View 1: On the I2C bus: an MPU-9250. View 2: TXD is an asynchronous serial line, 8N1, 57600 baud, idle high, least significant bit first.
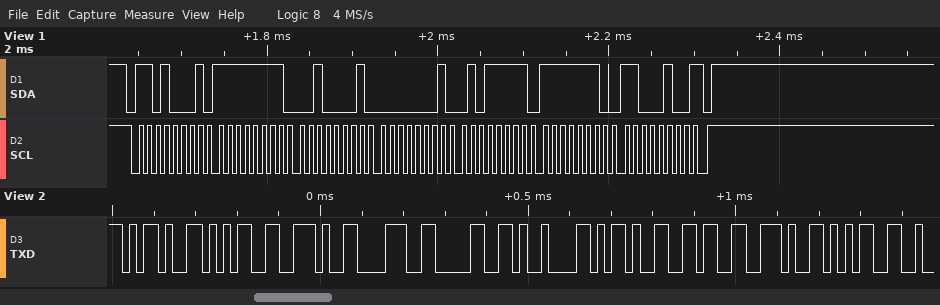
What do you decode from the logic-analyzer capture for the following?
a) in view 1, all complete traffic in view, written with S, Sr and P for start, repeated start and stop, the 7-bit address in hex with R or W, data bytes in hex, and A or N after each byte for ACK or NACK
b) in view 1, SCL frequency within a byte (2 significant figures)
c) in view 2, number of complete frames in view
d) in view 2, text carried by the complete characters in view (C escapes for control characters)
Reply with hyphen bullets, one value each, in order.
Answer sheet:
- S 68R A FF A 21 A 01 A 5F A FE A C4 N P
- 100 kHz
- 10
- "-5.80\t-6.5"
